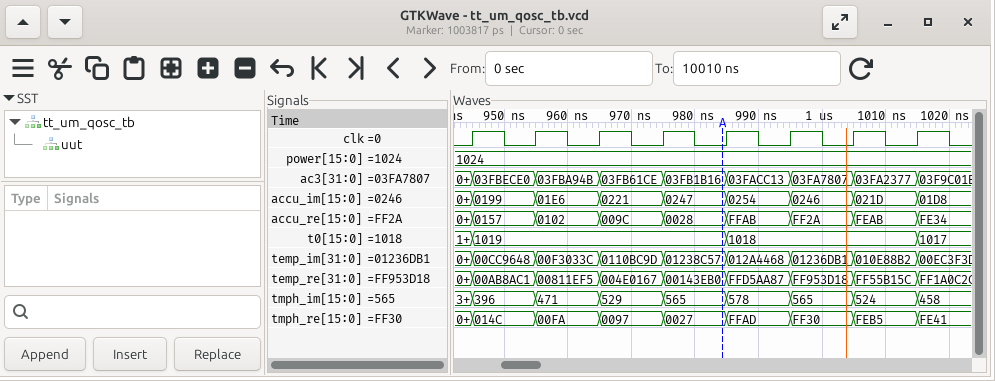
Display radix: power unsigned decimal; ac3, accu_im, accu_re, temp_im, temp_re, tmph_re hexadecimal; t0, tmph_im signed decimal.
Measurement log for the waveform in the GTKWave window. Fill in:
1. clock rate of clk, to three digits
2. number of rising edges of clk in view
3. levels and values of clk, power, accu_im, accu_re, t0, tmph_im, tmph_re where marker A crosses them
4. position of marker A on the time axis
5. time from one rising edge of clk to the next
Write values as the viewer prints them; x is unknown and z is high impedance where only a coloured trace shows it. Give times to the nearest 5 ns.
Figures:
100 MHz
8
clk=0, power=1024, accu_im=0247, accu_re=0028, t0=1019, tmph_im=565, tmph_re=0027
985 ns
10 ns
